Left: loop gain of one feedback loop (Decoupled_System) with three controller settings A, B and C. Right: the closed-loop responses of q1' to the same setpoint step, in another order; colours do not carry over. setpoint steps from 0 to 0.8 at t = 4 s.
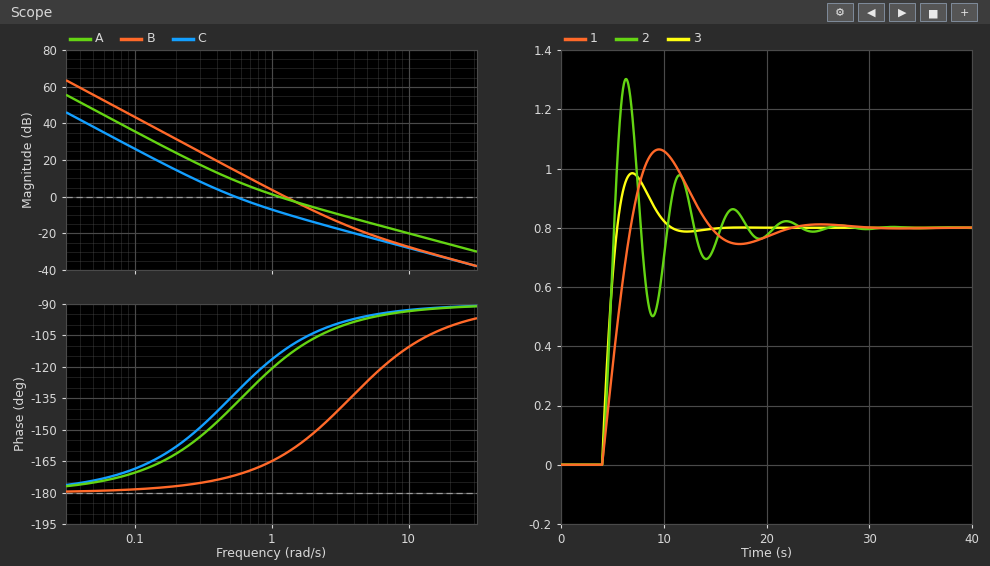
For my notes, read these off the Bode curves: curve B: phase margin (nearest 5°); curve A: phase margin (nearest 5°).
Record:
20°
60°
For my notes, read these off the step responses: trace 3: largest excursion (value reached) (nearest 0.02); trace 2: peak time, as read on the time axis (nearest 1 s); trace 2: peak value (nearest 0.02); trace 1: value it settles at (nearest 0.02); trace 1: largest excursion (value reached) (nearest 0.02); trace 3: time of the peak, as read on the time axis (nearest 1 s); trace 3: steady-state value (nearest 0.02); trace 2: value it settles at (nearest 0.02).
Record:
0.98
6 s
1.30
0.80
1.06
7 s
0.80
0.80
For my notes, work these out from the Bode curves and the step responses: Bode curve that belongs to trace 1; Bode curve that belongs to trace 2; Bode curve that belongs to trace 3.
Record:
C
B
A
